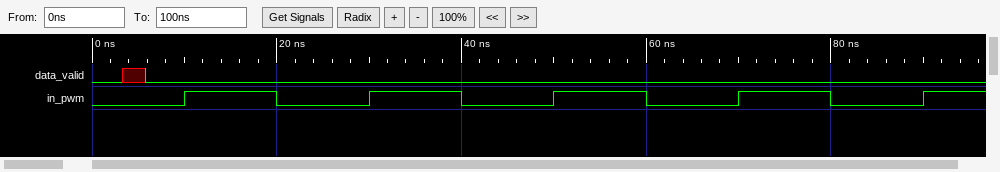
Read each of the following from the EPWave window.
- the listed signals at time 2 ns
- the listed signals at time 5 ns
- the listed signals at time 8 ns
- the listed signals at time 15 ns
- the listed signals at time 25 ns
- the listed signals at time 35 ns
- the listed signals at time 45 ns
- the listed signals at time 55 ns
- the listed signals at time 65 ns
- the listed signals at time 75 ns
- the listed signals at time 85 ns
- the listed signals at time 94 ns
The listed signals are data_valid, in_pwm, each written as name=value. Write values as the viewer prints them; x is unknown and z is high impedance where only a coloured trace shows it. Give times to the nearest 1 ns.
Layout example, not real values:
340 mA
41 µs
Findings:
data_valid=0, in_pwm=0
data_valid=x, in_pwm=0
data_valid=0, in_pwm=0
data_valid=0, in_pwm=1
data_valid=0, in_pwm=0
data_valid=0, in_pwm=1
data_valid=0, in_pwm=0
data_valid=0, in_pwm=1
data_valid=0, in_pwm=0
data_valid=0, in_pwm=1
data_valid=0, in_pwm=0
data_valid=0, in_pwm=1
